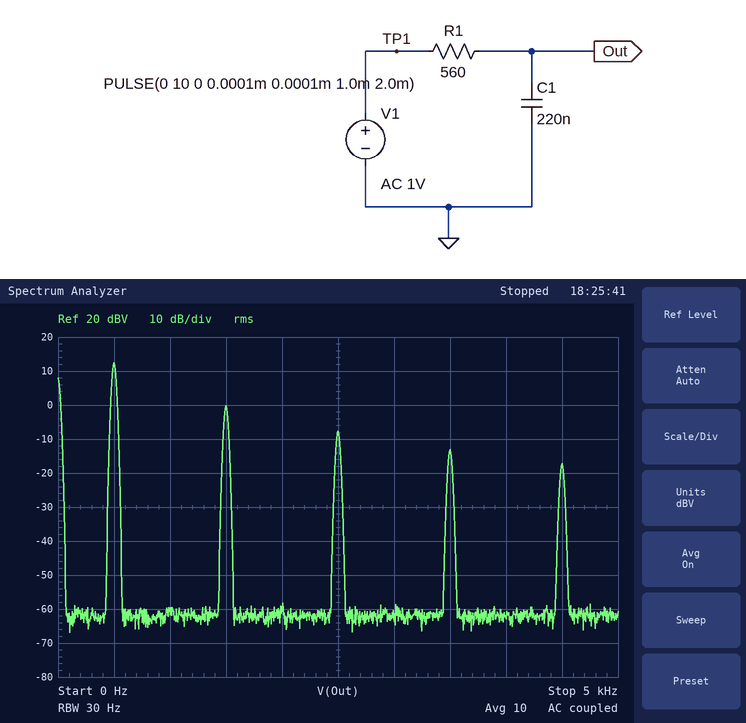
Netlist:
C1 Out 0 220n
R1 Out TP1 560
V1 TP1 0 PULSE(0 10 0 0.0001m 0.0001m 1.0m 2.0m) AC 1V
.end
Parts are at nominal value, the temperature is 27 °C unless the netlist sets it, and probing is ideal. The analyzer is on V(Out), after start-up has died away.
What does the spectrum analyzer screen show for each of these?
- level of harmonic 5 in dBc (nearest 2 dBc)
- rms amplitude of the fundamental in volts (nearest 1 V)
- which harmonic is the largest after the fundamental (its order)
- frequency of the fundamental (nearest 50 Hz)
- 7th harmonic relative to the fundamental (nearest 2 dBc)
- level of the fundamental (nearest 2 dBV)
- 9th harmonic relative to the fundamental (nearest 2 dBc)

-20 dBc
4 V
3
500 Hz
-26 dBc
12 dBV
-30 dBc
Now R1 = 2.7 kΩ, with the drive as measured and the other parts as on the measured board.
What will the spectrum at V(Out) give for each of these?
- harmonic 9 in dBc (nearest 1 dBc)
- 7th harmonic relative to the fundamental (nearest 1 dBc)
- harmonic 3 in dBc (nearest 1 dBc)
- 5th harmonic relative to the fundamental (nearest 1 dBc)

-37 dBc
-33 dBc
-18 dBc
-27 dBc
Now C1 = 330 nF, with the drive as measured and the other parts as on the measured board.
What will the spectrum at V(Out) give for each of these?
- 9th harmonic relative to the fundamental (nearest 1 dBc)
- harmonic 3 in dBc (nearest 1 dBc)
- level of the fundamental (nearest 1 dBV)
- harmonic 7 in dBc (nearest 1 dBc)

-32 dBc
-14 dBc
12 dBV
-28 dBc
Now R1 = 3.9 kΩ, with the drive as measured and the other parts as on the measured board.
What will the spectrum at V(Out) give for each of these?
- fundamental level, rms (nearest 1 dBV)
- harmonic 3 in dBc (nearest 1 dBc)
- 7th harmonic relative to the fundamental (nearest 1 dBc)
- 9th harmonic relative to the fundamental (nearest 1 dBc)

4 dBV
-19 dBc
-33 dBc
-38 dBc
